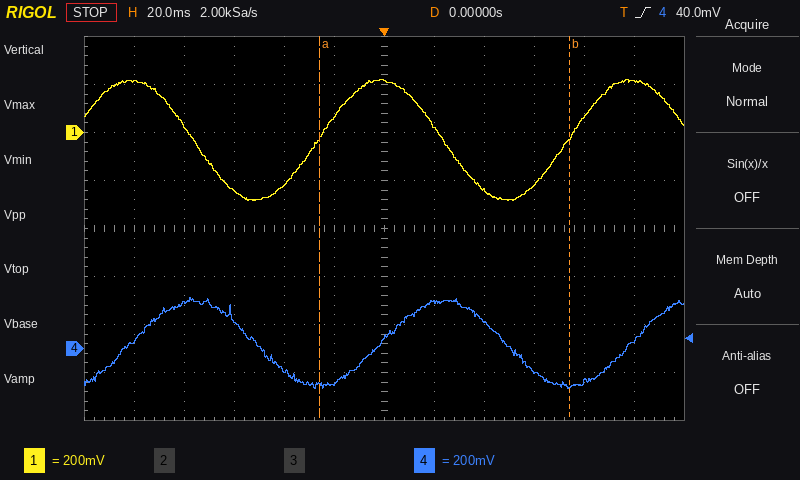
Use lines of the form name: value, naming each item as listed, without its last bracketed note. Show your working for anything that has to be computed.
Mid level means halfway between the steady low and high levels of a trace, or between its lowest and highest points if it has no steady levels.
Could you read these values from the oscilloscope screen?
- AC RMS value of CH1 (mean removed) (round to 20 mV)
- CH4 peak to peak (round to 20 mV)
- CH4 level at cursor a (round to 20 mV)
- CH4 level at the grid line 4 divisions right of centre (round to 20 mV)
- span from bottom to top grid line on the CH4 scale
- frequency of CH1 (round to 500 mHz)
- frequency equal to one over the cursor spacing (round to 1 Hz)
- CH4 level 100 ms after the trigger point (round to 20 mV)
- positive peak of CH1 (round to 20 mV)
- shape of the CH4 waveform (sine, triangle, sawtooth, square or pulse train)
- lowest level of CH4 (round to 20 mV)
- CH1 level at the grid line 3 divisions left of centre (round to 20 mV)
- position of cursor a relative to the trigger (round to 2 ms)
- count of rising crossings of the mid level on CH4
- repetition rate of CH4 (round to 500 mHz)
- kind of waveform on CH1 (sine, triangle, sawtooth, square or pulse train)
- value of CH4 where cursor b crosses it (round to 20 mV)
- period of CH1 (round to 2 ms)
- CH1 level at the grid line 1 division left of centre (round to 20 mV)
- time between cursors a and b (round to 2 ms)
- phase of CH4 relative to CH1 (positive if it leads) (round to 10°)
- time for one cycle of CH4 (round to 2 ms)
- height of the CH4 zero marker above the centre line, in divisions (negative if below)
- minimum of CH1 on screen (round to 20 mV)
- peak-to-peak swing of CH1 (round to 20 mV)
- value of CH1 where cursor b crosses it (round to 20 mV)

AC RMS value of CH1 (mean removed): 500 mV / (2√2) ≈ 177 mV, so 180 mV to the nearest 20 mV
CH4 peak to peak: 220 mV − (-160 mV) = 380 mV
CH4 level at cursor a: -160 mV
CH4 level at the grid line 4 divisions right of centre: -140 mV
span from bottom to top grid line on the CH4 scale: 1.6 V
frequency of CH1: 1 / 100 ms ≈ 10.0 Hz
frequency equal to one over the cursor spacing: 1 / 100 ms ≈ 10 Hz
CH4 level 100 ms after the trigger point: 40 mV
positive peak of CH1: 220 mV
shape of the CH4 waveform: sine
lowest level of CH4: -160 mV
CH1 level at the grid line 3 divisions left of centre: -240 mV
position of cursor a relative to the trigger: -26 ms
count of rising crossings of the mid level on CH4: 3
repetition rate of CH4: 1 / 100 ms ≈ 10.0 Hz
kind of waveform on CH1: sine
value of CH4 where cursor b crosses it: -160 mV
period of CH1: 100 ms
CH1 level at the grid line 1 division left of centre: 60 mV
time between cursors a and b: 100 ms
phase of CH4 relative to CH1 (positive if it leads): -90°
time for one cycle of CH4: 100 ms
height of the CH4 zero marker above the centre line, in divisions: -2.5 div
minimum of CH1 on screen: -280 mV
peak-to-peak swing of CH1: 220 mV − (-280 mV) = 500 mV
value of CH1 where cursor b crosses it: -20 mV
